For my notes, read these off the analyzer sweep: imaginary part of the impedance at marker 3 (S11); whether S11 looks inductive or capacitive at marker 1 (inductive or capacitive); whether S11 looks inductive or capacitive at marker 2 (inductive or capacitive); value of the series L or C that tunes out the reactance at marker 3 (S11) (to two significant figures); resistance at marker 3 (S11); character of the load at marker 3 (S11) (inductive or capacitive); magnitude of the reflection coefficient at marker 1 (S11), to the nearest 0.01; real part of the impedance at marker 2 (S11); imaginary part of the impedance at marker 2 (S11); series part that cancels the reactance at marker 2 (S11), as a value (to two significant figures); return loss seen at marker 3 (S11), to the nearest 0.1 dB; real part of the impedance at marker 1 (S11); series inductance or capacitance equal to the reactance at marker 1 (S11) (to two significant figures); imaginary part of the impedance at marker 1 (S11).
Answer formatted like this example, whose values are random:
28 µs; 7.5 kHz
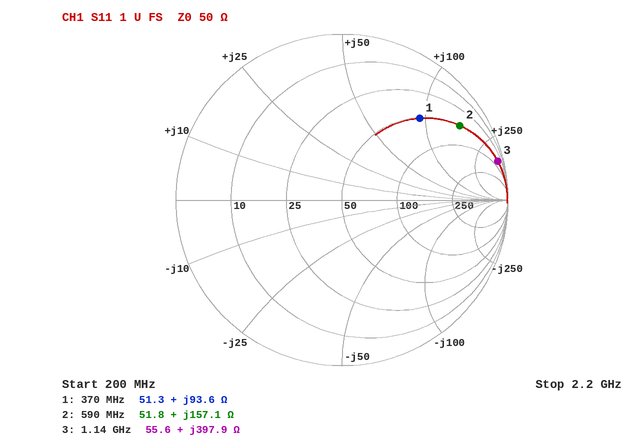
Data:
+397.9 Ω; inductive; inductive; 350 fF; 55.6 Ω; inductive; 0.68; 51.8 Ω; +157.1 Ω; 1.7 pF; 0.3 dB; 51.3 Ω; 40 nH; +93.6 Ω
